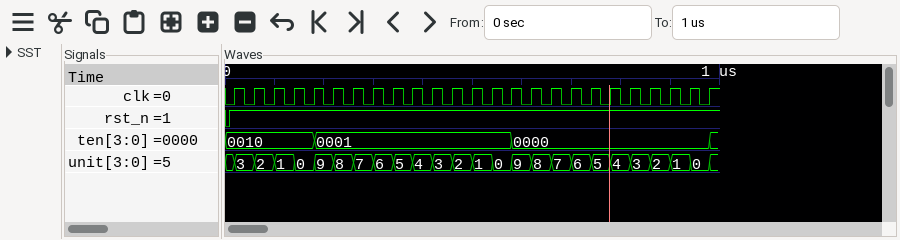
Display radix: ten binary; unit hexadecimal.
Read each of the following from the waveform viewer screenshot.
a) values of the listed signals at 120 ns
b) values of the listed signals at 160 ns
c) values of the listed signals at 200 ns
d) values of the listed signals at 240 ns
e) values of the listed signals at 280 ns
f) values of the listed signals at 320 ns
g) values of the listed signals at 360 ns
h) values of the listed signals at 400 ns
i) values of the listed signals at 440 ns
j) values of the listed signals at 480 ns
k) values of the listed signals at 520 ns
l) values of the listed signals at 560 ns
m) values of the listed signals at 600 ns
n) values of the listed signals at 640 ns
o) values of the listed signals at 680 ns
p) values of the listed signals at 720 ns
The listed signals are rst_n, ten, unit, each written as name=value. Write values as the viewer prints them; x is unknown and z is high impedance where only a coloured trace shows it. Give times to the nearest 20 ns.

rst_n=1, ten=0010, unit=1
rst_n=1, ten=0010, unit=0
rst_n=1, ten=0001, unit=9
rst_n=1, ten=0001, unit=8
rst_n=1, ten=0001, unit=7
rst_n=1, ten=0001, unit=6
rst_n=1, ten=0001, unit=5
rst_n=1, ten=0001, unit=4
rst_n=1, ten=0001, unit=3
rst_n=1, ten=0001, unit=2
rst_n=1, ten=0001, unit=1
rst_n=1, ten=0001, unit=0
rst_n=1, ten=0000, unit=9
rst_n=1, ten=0000, unit=8
rst_n=1, ten=0000, unit=7
rst_n=1, ten=0000, unit=6
